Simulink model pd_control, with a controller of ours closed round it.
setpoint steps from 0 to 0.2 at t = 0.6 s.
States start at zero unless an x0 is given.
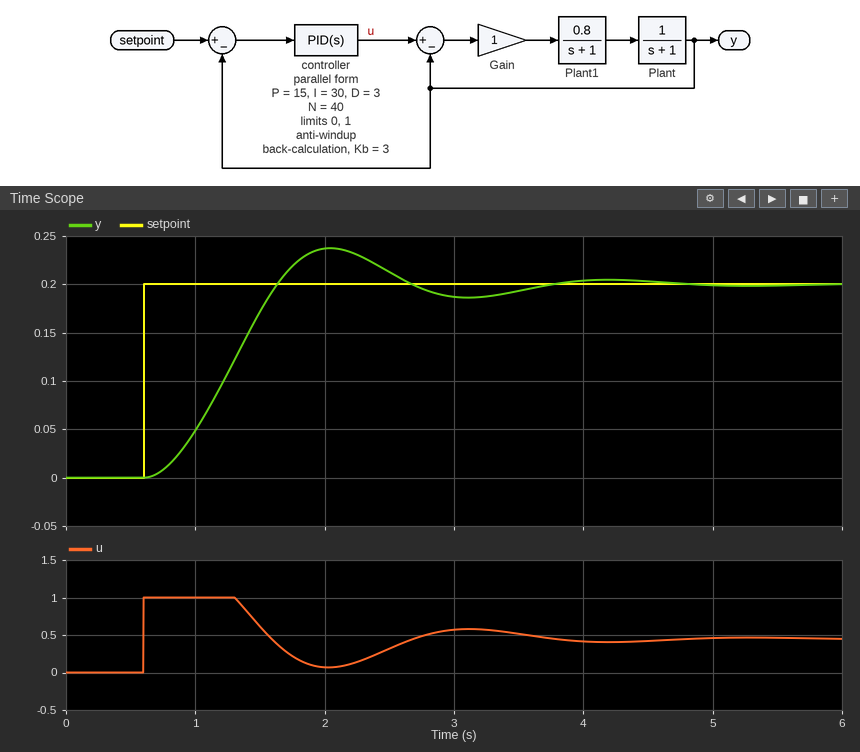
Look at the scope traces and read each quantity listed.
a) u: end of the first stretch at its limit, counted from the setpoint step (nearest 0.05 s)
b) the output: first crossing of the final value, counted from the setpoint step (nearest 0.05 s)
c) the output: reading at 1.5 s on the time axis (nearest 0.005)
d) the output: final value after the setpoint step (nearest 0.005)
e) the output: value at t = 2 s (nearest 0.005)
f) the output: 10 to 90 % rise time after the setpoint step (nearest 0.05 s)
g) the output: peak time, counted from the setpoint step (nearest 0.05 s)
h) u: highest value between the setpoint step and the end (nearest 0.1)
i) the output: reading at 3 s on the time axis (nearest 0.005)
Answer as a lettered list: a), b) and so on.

a) 0.70 s
b) 1.05 s
c) 0.170
d) 0.200
e) 0.235
f) 0.70 s
g) 1.45 s
h) 1.0
i) 0.185
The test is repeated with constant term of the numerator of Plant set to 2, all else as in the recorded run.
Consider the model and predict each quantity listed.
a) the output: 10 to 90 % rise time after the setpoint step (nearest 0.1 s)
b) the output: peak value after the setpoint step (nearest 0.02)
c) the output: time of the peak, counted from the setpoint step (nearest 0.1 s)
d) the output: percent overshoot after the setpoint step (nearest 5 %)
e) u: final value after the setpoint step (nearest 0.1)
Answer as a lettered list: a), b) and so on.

a) 0.5 s
b) 0.22
c) 1.1 s
d) 10 %
e) 0.3
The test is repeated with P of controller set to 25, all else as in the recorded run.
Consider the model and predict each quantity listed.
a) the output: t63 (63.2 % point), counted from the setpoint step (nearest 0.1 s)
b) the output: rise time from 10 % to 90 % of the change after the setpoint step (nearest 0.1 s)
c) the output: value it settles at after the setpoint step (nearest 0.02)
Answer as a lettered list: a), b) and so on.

a) 0.7 s
b) 0.8 s
c) 0.20
